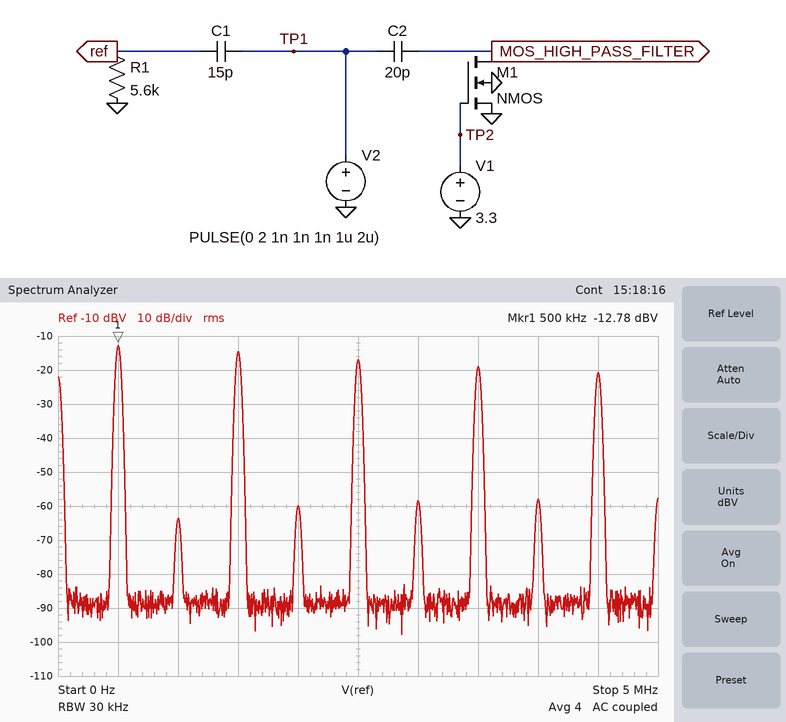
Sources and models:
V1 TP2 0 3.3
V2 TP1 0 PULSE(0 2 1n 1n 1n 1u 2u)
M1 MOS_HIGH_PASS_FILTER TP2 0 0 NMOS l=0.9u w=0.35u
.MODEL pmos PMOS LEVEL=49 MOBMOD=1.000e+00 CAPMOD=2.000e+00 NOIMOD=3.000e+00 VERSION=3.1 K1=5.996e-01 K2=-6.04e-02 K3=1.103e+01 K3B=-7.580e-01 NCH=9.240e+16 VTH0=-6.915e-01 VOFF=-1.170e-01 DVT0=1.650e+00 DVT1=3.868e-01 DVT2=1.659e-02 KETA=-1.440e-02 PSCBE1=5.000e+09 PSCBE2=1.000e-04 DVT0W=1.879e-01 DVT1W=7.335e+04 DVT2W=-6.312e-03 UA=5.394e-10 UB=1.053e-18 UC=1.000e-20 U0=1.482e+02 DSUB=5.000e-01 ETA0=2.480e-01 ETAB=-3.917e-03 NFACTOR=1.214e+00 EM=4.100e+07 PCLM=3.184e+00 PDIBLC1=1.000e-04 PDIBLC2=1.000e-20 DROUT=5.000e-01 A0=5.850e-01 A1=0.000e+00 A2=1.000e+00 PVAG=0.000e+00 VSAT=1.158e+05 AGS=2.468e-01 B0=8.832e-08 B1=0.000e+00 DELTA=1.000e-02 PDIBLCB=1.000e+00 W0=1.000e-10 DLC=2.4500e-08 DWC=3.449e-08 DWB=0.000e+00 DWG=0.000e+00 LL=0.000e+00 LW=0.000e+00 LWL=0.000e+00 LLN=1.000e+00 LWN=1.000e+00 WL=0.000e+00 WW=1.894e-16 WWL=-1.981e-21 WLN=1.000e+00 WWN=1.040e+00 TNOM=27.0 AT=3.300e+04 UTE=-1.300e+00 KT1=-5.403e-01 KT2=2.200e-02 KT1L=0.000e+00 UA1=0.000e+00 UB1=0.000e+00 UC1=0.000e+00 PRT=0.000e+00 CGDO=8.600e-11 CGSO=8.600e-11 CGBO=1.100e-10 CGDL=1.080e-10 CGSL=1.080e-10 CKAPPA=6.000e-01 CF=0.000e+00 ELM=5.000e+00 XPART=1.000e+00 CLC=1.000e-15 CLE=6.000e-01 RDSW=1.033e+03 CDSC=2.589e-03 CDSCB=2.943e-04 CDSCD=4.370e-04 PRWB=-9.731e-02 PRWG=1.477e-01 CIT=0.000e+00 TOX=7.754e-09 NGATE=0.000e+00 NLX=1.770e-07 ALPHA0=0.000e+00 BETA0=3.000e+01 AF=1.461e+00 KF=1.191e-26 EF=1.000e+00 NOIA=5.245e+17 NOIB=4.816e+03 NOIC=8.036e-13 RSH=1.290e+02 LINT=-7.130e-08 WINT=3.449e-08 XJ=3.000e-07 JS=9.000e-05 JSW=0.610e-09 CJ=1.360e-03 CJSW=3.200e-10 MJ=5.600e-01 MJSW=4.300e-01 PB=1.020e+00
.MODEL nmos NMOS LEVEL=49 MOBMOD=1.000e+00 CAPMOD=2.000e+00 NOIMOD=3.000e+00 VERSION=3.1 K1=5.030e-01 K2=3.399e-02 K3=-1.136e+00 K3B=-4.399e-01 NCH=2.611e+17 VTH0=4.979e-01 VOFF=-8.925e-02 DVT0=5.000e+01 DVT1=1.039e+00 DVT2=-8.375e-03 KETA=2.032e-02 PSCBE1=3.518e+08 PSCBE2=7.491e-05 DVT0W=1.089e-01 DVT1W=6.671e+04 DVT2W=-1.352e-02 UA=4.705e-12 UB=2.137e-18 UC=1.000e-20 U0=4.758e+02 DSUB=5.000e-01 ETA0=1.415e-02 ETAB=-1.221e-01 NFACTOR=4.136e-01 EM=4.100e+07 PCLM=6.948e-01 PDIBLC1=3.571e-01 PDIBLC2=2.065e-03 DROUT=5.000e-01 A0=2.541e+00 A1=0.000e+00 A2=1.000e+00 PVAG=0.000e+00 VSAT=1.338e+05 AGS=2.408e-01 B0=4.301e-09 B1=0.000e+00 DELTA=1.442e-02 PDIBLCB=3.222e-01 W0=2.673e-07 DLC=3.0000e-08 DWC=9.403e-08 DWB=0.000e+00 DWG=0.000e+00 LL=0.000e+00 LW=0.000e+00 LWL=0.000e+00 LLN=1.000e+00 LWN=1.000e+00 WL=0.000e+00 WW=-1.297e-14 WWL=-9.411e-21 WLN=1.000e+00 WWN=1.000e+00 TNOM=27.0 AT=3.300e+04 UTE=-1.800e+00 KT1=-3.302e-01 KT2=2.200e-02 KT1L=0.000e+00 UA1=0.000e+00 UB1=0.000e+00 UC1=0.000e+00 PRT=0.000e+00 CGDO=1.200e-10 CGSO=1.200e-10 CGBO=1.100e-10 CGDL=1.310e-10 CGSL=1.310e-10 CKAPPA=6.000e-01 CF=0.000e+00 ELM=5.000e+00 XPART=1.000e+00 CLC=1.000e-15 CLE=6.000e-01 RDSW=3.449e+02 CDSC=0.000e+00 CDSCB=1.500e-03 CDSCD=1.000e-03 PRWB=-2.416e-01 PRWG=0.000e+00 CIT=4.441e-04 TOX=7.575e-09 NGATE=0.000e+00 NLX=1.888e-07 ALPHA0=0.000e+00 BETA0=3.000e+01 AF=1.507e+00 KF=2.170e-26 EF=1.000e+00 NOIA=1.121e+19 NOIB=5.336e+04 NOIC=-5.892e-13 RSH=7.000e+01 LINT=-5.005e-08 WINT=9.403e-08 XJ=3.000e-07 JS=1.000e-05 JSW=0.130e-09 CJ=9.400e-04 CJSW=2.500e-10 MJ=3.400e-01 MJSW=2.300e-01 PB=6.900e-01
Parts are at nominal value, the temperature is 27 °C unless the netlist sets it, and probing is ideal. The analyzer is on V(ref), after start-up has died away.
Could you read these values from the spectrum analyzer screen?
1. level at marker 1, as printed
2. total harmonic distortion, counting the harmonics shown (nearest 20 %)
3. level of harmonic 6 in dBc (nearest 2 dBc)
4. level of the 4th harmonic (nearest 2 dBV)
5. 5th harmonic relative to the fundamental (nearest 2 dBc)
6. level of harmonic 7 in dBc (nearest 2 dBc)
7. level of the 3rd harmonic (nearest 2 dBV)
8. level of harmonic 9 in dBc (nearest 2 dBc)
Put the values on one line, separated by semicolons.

-12.78 dBV; 120 %; -46 dBc; -60 dBV; -4 dBc; -6 dBc; -14 dBV; -8 dBc
